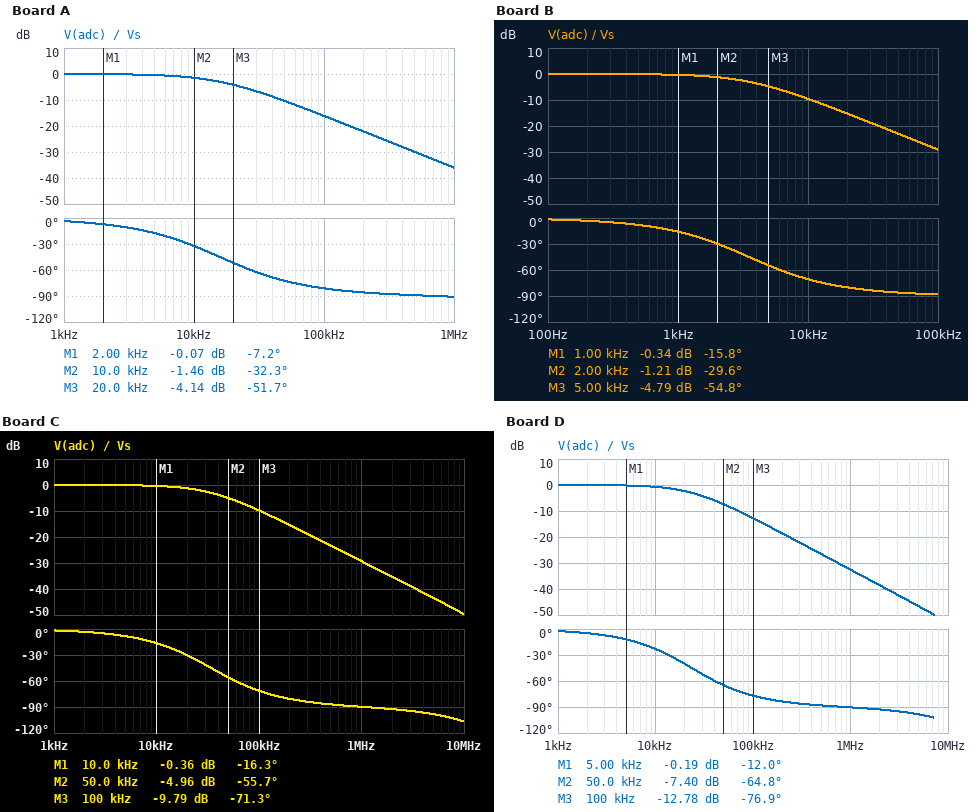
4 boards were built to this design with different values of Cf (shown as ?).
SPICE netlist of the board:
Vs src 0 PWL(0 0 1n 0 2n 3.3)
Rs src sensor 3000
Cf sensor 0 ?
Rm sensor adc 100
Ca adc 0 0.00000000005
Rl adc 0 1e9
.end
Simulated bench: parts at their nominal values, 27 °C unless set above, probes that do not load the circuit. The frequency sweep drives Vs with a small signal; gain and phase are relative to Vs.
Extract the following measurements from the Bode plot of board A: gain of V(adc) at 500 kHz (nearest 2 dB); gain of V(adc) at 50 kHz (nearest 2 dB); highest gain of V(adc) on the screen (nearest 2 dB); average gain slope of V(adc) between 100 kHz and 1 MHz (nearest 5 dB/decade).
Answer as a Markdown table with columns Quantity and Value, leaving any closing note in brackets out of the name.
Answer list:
| Quantity | Value |
|---|---|
| gain of V(adc) at 500 kHz | -30 dB |
| gain of V(adc) at 50 kHz | -10 dB |
| highest gain of V(adc) on the screen | 0 dB |
| average gain slope of V(adc) between 100 kHz and 1 MHz | -20 dB/decade |
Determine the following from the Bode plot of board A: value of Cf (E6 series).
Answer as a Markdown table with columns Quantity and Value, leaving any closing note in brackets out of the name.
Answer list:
| Quantity | Value |
|---|---|
| value of Cf | 3.3 nF |
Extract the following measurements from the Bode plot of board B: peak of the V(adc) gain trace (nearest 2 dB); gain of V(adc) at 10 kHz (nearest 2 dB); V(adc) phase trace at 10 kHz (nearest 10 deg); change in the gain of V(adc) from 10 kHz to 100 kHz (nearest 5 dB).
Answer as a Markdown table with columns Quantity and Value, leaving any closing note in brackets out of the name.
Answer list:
| Quantity | Value |
|---|---|
| peak of the V(adc) gain trace | 0 dB |
| gain of V(adc) at 10 kHz | -10 dB |
| V(adc) phase trace at 10 kHz | -70 deg |
| change in the gain of V(adc) from 10 kHz to 100 kHz | -20 dB |
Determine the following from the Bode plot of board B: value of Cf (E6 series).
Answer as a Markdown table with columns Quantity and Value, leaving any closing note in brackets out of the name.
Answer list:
| Quantity | Value |
|---|---|
| value of Cf | 15 nF |
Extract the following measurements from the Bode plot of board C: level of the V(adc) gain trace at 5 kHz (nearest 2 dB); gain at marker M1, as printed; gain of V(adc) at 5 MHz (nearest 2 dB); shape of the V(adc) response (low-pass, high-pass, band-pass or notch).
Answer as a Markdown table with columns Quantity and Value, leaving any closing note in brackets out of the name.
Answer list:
| Quantity | Value |
|---|---|
| level of the V(adc) gain trace at 5 kHz | 0 dB |
| gain at marker M1, as printed | -0.36 dB |
| gain of V(adc) at 5 MHz | -44 dB |
| shape of the V(adc) response | low-pass |
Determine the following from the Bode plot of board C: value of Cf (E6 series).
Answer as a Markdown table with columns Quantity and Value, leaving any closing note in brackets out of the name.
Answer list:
| Quantity | Value |
|---|---|
| value of Cf | 1.5 nF |
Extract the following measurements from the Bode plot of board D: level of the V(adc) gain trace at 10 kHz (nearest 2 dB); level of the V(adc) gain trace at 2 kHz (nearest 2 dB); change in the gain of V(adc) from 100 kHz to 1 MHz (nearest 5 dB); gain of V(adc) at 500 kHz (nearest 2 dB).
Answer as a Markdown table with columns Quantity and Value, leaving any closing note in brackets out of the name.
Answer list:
| Quantity | Value |
|---|---|
| level of the V(adc) gain trace at 10 kHz | 0 dB |
| level of the V(adc) gain trace at 2 kHz | 0 dB |
| change in the gain of V(adc) from 100 kHz to 1 MHz | -20 dB |
| gain of V(adc) at 500 kHz | -26 dB |
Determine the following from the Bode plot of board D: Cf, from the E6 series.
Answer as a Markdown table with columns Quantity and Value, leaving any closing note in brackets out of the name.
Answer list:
| Quantity | Value |
|---|---|
| Cf, from the E6 series | 2.2 nF |
